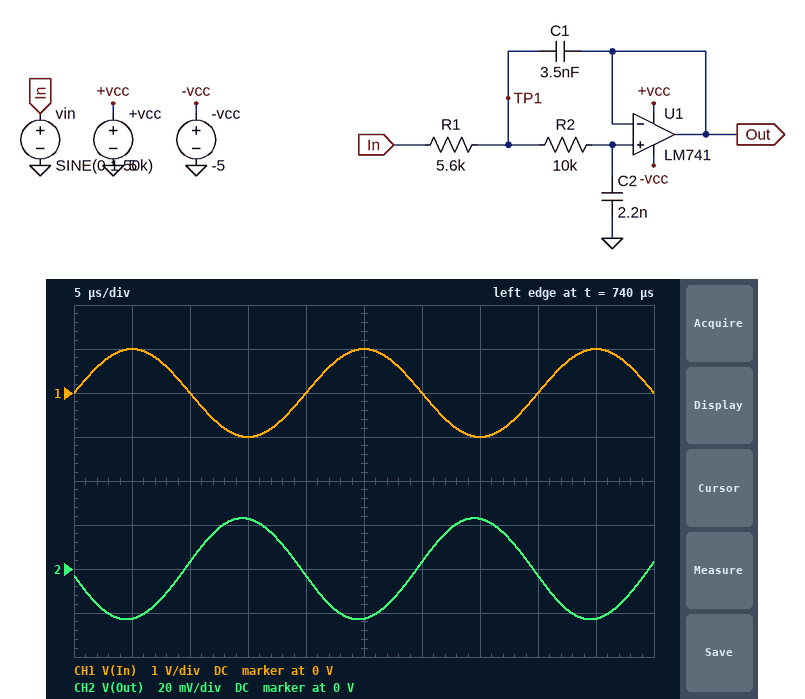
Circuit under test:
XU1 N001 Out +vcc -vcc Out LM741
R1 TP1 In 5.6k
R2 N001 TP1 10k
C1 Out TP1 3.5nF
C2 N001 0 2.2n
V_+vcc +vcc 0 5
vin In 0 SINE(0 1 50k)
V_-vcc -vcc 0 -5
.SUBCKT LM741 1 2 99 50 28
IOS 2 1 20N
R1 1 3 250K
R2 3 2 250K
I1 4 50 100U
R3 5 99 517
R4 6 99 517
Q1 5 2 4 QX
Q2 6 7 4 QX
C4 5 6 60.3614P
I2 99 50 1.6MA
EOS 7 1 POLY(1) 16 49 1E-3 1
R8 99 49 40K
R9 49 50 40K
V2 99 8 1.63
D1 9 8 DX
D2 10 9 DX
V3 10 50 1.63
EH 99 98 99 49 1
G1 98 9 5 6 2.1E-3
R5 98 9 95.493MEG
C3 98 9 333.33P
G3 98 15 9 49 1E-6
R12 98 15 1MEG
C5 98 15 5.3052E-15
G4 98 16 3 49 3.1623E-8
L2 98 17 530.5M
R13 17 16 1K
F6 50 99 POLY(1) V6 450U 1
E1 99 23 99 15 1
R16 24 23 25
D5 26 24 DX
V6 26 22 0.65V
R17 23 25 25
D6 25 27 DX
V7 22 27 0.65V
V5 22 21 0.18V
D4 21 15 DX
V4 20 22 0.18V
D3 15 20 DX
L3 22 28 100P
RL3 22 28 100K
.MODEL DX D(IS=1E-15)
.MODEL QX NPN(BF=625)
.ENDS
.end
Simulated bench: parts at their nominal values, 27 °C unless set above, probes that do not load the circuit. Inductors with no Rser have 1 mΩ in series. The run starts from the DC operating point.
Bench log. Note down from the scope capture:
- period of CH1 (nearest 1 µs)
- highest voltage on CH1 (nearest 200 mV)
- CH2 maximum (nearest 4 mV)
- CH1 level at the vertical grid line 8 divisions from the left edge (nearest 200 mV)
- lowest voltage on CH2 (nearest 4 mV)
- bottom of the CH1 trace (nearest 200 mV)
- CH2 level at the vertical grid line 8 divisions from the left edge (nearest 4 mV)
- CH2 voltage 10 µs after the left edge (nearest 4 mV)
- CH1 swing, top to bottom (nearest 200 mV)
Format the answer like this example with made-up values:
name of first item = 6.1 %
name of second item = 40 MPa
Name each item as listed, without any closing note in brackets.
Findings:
period of CH1 = 20 µs
highest voltage on CH1 = 1.0 V
CH2 maximum = 24 mV
CH1 level at the vertical grid line 8 divisions from the left edge = 0 V
lowest voltage on CH2 = -24 mV
bottom of the CH1 trace = -1.0 V
CH2 level at the vertical grid line 8 divisions from the left edge = -4 mV
CH2 voltage 10 µs after the left edge = 4 mV
CH1 swing, top to bottom = 2.0 V
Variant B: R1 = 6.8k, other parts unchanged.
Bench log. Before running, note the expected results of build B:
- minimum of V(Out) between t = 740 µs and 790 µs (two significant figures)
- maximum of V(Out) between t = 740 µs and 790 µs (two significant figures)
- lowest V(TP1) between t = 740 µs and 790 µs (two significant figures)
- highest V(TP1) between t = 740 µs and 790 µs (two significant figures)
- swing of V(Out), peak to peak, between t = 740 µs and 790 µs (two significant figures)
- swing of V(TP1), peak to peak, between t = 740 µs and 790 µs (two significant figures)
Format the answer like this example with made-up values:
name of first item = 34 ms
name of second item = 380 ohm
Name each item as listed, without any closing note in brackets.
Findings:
minimum of V(Out) between t = 740 µs and 790 µs = -19 mV
maximum of V(Out) between t = 740 µs and 790 µs = 19 mV
lowest V(TP1) between t = 740 µs and 790 µs = -130 mV
highest V(TP1) between t = 740 µs and 790 µs = 130 mV
swing of V(Out), peak to peak, between t = 740 µs and 790 µs = 38 mV
swing of V(TP1), peak to peak, between t = 740 µs and 790 µs = 260 mV
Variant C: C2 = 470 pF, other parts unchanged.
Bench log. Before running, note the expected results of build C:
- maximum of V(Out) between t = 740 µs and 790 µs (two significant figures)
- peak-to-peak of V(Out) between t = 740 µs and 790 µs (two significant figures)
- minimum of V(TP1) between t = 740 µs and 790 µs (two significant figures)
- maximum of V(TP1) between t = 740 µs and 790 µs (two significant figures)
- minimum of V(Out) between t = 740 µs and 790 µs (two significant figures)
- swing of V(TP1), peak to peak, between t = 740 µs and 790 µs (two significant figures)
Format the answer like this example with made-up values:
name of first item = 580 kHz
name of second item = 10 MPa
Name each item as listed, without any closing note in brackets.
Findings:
maximum of V(Out) between t = 740 µs and 790 µs = 110 mV
peak-to-peak of V(Out) between t = 740 µs and 790 µs = 230 mV
minimum of V(TP1) between t = 740 µs and 790 µs = -200 mV
maximum of V(TP1) between t = 740 µs and 790 µs = 200 mV
minimum of V(Out) between t = 740 µs and 790 µs = -110 mV
swing of V(TP1), peak to peak, between t = 740 µs and 790 µs = 410 mV
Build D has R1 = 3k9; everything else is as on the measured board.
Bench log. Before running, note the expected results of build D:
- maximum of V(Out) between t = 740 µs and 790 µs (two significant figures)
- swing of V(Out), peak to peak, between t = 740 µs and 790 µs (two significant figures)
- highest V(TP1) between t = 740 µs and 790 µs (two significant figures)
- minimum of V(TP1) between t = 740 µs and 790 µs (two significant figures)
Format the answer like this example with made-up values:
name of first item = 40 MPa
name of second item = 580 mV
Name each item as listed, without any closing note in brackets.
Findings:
maximum of V(Out) between t = 740 µs and 790 µs = 33 mV
swing of V(Out), peak to peak, between t = 740 µs and 790 µs = 65 mV
highest V(TP1) between t = 740 µs and 790 µs = 230 mV
minimum of V(TP1) between t = 740 µs and 790 µs = -230 mV
